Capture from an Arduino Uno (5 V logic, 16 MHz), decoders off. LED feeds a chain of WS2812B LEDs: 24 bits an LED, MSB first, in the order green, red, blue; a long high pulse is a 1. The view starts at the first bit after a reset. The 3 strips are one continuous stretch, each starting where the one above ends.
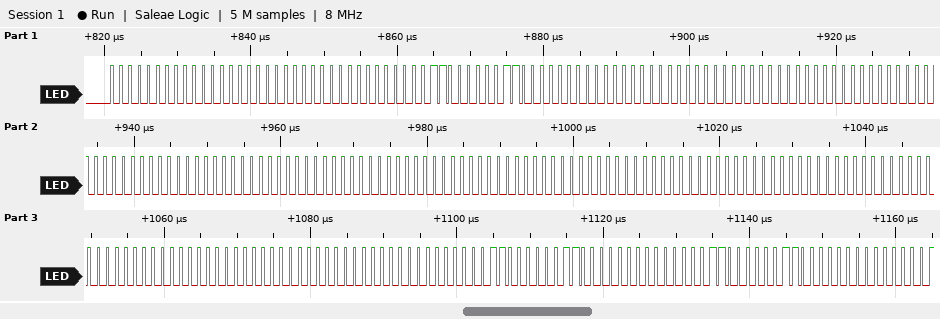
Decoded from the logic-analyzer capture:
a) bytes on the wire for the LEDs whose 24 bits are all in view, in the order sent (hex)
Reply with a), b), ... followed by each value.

a) 00 00 00 00 18 18 00 00 00 00 00 00 00 00 00 00 00 00 00 00 00 00 00 00 00 00 00 00 18 18 00 18 18
